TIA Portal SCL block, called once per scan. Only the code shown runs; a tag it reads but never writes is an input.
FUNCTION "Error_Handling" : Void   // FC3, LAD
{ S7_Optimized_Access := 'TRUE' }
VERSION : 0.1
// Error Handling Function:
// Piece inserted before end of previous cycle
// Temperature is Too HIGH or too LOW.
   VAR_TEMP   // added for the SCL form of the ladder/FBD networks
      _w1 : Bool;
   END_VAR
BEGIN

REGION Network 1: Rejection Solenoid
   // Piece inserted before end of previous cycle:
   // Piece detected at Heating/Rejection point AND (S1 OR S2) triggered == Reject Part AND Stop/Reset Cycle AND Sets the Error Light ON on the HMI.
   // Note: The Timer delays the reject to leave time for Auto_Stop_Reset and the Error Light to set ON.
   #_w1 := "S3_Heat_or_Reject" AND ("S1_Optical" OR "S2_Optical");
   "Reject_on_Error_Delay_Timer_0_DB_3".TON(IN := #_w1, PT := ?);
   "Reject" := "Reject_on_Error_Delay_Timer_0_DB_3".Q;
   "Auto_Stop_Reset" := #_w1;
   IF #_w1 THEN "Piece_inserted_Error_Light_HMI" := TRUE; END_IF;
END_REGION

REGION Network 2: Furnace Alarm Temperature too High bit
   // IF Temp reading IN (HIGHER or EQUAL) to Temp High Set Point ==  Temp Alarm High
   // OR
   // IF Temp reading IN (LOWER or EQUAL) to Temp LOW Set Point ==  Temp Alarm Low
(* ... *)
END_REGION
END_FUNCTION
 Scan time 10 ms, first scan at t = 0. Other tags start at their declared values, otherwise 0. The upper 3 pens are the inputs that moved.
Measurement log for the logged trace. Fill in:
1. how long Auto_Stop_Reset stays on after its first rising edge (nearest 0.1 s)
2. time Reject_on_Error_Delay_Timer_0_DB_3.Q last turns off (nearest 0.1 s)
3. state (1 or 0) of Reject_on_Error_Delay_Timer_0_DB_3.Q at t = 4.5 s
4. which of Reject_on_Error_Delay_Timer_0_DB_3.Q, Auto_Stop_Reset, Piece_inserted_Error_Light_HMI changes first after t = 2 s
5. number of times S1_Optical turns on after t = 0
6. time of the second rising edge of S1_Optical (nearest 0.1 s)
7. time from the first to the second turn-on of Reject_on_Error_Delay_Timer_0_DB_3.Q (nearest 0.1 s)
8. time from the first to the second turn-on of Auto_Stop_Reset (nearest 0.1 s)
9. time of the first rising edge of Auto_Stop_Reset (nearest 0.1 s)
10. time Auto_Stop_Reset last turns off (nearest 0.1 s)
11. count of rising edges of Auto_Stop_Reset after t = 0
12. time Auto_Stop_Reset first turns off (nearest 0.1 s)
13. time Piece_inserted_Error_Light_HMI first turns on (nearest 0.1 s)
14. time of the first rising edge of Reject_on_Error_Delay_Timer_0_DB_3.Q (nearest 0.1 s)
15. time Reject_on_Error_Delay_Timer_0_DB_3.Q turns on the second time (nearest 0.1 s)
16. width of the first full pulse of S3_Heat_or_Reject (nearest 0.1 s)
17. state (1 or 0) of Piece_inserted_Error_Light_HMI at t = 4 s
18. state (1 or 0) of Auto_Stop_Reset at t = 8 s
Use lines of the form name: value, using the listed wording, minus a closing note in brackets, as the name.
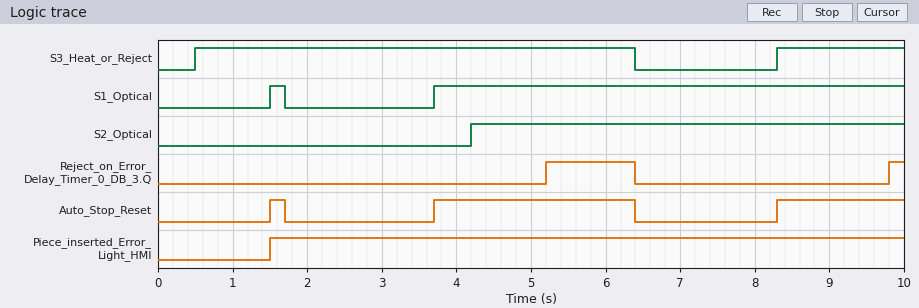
how long Auto_Stop_Reset stays on after its first rising edge: 0.2 s
time Reject_on_Error_Delay_Timer_0_DB_3.Q last turns off: 6.4 s
state (1 or 0) of Reject_on_Error_Delay_Timer_0_DB_3.Q at t = 4.5 s: 0
which of Reject_on_Error_Delay_Timer_0_DB_3.Q, Auto_Stop_Reset, Piece_inserted_Error_Light_HMI changes first after t = 2 s: Auto_Stop_Reset
number of times S1_Optical turns on after t = 0: 2
time of the second rising edge of S1_Optical: 3.7 s
time from the first to the second turn-on of Reject_on_Error_Delay_Timer_0_DB_3.Q: 4.6 s
time from the first to the second turn-on of Auto_Stop_Reset: 2.2 s
time of the first rising edge of Auto_Stop_Reset: 1.5 s
time Auto_Stop_Reset last turns off: 6.4 s
count of rising edges of Auto_Stop_Reset after t = 0: 3
time Auto_Stop_Reset first turns off: 1.7 s
time Piece_inserted_Error_Light_HMI first turns on: 1.5 s
time of the first rising edge of Reject_on_Error_Delay_Timer_0_DB_3.Q: 5.2 s
time Reject_on_Error_Delay_Timer_0_DB_3.Q turns on the second time: 9.8 s
width of the first full pulse of S3_Heat_or_Reject: 5.9 s
state (1 or 0) of Piece_inserted_Error_Light_HMI at t = 4 s: 1
state (1 or 0) of Auto_Stop_Reset at t = 8 s: 0
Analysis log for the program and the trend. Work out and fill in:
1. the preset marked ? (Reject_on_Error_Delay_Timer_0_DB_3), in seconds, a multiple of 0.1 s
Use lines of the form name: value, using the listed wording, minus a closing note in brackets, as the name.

the preset marked ? (Reject_on_Error_Delay_Timer_0_DB_3), in seconds, a multiple of 0.1 s: 1.5 s
